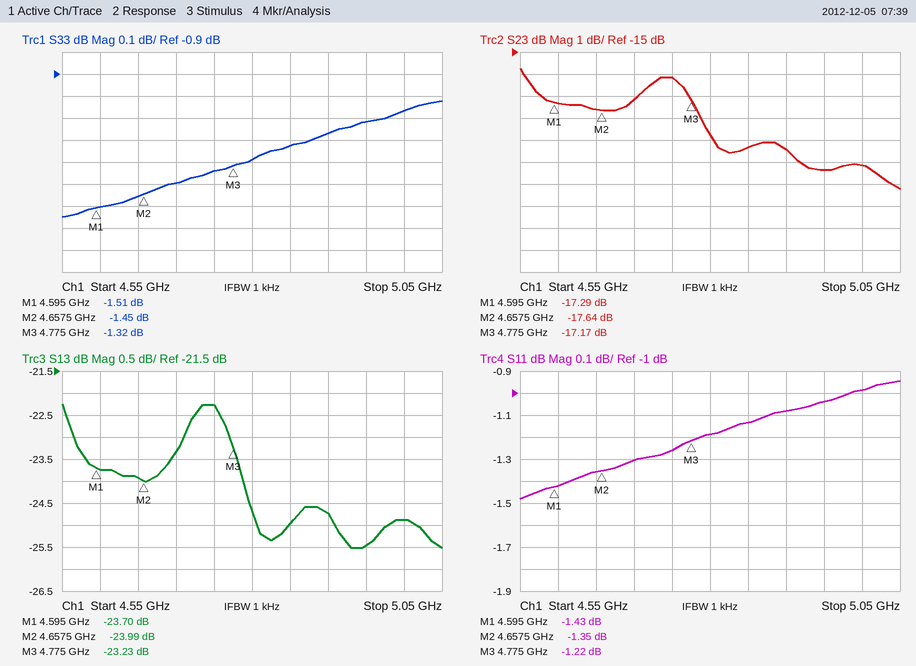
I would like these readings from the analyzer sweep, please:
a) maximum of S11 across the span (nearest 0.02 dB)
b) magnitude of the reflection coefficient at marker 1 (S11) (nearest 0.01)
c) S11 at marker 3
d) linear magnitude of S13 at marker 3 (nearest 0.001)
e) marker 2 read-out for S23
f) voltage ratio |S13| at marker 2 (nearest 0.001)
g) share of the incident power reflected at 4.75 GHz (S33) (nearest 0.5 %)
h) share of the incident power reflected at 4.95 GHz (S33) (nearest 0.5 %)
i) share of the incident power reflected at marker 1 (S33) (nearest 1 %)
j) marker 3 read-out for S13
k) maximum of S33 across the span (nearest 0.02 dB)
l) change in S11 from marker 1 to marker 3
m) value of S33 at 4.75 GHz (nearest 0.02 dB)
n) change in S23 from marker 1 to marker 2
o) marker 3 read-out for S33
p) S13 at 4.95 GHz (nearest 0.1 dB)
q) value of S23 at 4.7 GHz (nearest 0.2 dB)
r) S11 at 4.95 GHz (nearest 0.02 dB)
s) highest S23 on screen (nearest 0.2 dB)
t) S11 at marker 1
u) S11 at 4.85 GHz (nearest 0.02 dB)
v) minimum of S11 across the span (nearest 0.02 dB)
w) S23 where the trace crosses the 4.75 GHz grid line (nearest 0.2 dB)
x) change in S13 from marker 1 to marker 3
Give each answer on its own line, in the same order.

-0.94 dB
0.85
-1.22 dB
0.069
-17.64 dB
0.063
73.5 %
77.5 %
71 %
-23.23 dB
-1.02 dB
0.21 dB
-1.34 dB
-0.35 dB
-1.32 dB
-25.5 dB
-17.2 dB
-1.04 dB
-15.8 dB
-1.43 dB
-1.14 dB
-1.48 dB
-16.2 dB
0.47 dB
